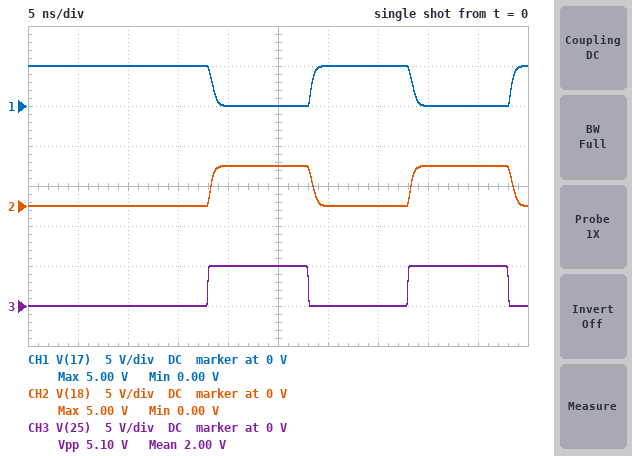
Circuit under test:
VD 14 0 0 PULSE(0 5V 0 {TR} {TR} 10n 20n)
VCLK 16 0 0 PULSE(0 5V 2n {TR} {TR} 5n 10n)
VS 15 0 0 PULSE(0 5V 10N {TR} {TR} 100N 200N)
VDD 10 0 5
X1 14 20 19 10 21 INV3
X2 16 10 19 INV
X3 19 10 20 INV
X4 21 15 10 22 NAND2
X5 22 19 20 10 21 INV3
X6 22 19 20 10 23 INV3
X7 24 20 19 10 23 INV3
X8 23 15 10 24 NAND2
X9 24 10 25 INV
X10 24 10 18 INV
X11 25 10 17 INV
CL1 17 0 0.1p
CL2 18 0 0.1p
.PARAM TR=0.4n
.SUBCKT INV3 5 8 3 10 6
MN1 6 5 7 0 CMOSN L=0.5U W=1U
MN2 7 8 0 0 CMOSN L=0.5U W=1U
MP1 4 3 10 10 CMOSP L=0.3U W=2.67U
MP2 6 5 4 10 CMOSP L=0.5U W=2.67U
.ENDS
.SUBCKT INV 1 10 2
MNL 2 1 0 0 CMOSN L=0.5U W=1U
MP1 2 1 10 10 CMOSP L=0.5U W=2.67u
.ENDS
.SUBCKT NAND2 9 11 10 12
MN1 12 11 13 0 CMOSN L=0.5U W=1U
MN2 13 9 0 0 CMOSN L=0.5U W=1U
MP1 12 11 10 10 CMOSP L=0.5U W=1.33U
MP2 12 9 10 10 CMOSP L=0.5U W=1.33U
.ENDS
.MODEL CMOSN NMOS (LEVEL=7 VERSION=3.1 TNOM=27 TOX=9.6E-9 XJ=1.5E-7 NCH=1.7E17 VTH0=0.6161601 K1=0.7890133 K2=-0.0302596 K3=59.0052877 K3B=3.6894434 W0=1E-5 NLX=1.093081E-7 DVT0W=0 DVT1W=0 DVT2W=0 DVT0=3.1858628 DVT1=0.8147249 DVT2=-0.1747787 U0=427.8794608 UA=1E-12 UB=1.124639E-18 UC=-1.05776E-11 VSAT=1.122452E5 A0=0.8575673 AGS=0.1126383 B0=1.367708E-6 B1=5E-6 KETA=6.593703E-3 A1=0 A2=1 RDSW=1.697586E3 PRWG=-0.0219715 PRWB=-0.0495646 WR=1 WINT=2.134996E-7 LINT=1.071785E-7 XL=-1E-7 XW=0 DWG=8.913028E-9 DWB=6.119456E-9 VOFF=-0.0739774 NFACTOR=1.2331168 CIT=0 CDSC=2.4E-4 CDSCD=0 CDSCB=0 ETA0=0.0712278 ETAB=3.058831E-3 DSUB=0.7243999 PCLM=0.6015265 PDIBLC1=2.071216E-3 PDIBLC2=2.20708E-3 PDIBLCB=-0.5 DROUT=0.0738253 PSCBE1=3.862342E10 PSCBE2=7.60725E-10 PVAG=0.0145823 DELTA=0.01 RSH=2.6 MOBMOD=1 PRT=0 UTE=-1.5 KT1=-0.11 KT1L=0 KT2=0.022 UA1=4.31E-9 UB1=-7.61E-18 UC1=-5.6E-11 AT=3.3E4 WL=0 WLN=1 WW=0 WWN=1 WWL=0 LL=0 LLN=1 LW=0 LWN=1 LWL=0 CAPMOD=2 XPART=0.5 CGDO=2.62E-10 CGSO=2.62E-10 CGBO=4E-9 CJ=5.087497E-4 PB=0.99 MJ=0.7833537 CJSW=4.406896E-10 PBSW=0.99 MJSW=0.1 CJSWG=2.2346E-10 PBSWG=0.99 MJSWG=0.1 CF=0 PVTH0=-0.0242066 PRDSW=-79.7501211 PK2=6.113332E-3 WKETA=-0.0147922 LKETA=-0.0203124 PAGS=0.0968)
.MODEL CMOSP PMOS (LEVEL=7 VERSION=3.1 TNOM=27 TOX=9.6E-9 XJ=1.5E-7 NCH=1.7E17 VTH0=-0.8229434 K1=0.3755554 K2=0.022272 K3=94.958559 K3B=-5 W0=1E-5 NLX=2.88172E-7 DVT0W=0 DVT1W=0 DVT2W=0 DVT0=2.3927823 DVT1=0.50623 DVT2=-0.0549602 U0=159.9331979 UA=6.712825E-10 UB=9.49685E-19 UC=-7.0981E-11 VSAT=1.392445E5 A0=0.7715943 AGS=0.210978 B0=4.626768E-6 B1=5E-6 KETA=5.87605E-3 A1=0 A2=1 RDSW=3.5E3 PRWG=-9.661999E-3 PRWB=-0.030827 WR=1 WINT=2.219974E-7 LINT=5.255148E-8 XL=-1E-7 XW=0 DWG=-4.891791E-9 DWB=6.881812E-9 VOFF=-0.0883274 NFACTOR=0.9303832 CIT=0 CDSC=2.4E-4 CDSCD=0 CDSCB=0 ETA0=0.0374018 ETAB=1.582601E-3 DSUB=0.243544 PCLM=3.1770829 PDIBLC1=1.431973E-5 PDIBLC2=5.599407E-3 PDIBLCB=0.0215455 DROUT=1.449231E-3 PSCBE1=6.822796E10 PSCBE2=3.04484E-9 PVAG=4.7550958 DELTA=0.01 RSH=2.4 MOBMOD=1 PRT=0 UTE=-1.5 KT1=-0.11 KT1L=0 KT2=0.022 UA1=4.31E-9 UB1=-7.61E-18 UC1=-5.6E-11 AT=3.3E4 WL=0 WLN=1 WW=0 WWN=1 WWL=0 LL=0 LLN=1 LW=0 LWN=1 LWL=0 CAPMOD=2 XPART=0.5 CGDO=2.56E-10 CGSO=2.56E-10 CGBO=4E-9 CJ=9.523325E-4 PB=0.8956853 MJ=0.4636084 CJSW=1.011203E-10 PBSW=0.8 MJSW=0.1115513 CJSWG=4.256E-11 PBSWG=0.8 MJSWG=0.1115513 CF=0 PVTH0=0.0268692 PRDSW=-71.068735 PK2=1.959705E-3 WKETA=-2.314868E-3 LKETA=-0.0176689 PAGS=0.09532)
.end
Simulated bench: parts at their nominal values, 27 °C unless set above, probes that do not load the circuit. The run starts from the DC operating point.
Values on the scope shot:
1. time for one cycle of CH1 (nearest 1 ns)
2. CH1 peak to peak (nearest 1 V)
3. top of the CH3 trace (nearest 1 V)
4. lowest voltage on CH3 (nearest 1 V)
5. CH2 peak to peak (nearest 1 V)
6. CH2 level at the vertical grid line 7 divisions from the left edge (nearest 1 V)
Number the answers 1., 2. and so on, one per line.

1. 20 ns
2. 5 V
3. 5 V
4. 0 V
5. 5 V
6. 0 V
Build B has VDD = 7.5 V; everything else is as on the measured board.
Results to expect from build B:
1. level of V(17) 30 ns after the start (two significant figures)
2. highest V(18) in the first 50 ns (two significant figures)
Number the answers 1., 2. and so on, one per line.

1. 7.5 V
2. 7.4 V
